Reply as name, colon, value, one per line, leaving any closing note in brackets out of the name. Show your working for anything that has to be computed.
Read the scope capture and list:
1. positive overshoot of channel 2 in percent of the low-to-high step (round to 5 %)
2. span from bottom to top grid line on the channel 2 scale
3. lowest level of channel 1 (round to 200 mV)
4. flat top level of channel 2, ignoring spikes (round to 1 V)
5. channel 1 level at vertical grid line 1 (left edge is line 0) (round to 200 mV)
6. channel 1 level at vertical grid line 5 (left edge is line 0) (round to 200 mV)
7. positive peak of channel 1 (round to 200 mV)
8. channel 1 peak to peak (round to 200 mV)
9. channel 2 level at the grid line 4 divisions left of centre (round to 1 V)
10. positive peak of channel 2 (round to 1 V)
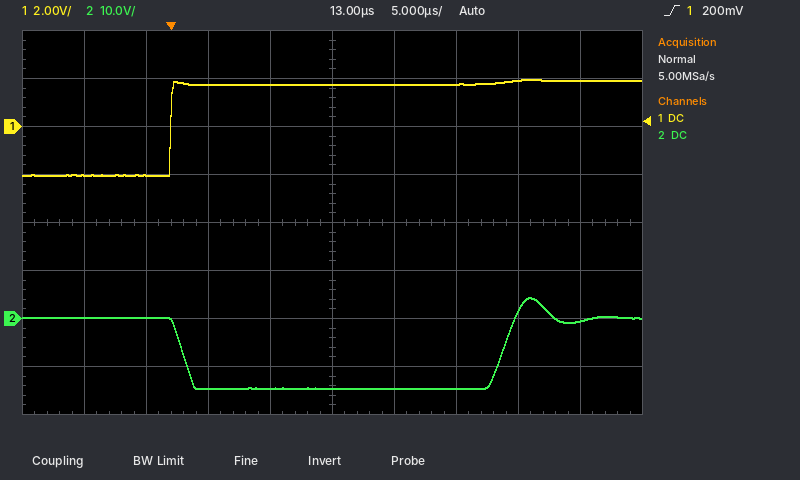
positive overshoot of channel 2 in percent of the low-to-high step: 30 %
span from bottom to top grid line on the channel 2 scale: 80 V
lowest level of channel 1: -2.0 V
flat top level of channel 2, ignoring spikes: 0 V
channel 1 level at vertical grid line 1 (left edge is line 0): -2.0 V
channel 1 level at vertical grid line 5 (left edge is line 0): 1.8 V
positive peak of channel 1: 2.0 V
channel 1 peak to peak: 2.0 V − (-2.0 V) = 4.0 V
channel 2 level at the grid line 4 divisions left of centre: 0 V
positive peak of channel 2: 4 V
